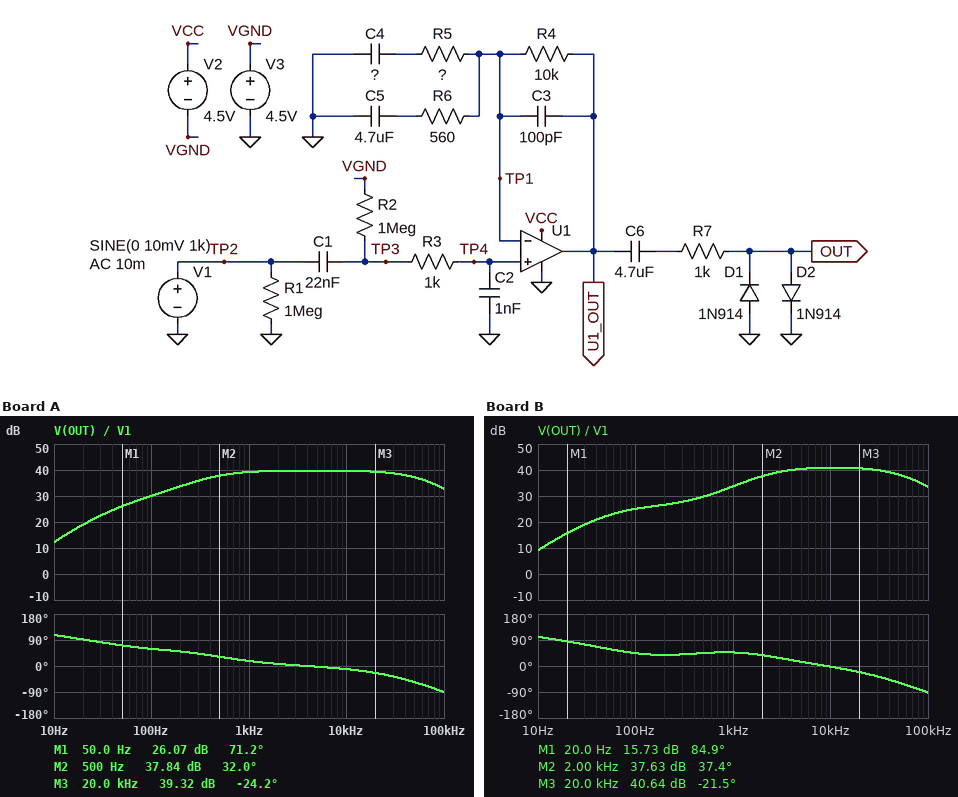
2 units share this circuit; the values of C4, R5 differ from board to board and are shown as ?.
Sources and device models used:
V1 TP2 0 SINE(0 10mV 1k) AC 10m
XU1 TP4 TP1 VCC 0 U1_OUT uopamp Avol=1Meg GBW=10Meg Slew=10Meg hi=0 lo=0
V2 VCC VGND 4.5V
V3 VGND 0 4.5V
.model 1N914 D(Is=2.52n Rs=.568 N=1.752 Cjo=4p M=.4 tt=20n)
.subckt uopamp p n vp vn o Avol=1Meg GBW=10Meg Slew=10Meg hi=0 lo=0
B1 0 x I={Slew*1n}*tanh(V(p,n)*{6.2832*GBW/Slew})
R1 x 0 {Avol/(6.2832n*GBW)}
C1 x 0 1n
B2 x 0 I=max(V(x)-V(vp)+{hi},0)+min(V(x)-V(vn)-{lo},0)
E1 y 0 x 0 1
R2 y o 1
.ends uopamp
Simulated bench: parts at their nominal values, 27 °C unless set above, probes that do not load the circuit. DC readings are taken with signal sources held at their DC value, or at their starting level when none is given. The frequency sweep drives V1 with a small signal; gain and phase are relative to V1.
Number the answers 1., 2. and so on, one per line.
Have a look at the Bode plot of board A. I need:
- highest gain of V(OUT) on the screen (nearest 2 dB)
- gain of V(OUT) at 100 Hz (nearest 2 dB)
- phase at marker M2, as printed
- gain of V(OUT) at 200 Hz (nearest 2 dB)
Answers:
1. 40 dB
2. 30 dB
3. 32.0 deg
4. 34 dB
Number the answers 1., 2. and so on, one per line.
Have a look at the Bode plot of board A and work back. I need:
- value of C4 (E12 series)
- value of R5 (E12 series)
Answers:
1. 3.3 µF
2. 120 Ω
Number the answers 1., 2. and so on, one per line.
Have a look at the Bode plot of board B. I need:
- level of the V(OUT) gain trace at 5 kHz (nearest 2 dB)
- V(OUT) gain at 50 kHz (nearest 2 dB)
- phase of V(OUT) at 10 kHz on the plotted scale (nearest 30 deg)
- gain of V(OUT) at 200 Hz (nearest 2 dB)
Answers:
1. 40 dB
2. 38 dB
3. 0 deg
4. 26 dB
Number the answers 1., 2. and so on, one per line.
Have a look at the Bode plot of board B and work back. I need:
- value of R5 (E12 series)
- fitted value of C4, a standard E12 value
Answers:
1. 100 Ω
2. 680 nF
